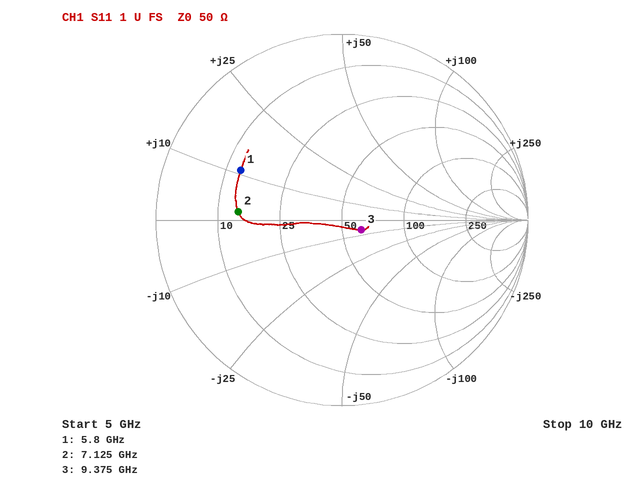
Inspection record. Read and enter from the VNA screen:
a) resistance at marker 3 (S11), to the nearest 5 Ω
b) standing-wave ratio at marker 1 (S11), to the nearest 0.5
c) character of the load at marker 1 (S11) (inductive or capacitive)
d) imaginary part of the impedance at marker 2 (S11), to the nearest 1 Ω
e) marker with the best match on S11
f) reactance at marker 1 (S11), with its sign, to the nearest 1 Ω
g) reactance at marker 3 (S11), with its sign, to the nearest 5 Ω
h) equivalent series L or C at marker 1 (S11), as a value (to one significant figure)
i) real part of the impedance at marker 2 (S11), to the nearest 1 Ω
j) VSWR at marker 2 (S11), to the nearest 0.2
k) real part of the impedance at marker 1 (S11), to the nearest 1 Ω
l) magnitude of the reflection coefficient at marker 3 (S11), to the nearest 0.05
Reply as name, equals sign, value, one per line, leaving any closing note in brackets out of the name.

resistance at marker 3 (S11), to the nearest 5 Ω = 60 Ω
standing-wave ratio at marker 1 (S11), to the nearest 0.5 = 4.0
character of the load at marker 1 (S11) = inductive
imaginary part of the impedance at marker 2 (S11), to the nearest 1 Ω = +2 Ω
marker with the best match on S11 = marker 3
reactance at marker 1 (S11), with its sign, to the nearest 1 Ω = +11 Ω
reactance at marker 3 (S11), with its sign, to the nearest 5 Ω = -5 Ω
equivalent series L or C at marker 1 (S11), as a value = 300 pH
real part of the impedance at marker 2 (S11), to the nearest 1 Ω = 14 Ω
VSWR at marker 2 (S11), to the nearest 0.2 = 3.6
real part of the impedance at marker 1 (S11), to the nearest 1 Ω = 13 Ω
magnitude of the reflection coefficient at marker 3 (S11), to the nearest 0.05 = 0.10
